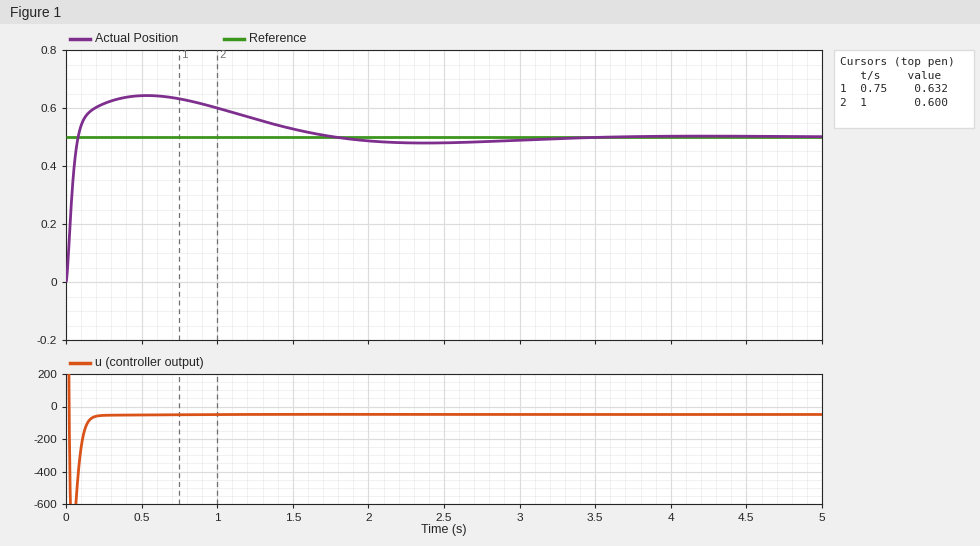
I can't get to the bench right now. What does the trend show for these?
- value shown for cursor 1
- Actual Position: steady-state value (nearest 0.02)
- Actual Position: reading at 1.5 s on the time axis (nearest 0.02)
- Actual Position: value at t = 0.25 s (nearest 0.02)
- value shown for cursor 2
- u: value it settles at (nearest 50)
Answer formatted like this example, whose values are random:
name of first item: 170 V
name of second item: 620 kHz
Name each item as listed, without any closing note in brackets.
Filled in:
value shown for cursor 1: 0.632
Actual Position: steady-state value: 0.50
Actual Position: reading at 1.5 s on the time axis: 0.52
Actual Position: value at t = 0.25 s: 0.62
value shown for cursor 2: 0.600
u: value it settles at: -50
